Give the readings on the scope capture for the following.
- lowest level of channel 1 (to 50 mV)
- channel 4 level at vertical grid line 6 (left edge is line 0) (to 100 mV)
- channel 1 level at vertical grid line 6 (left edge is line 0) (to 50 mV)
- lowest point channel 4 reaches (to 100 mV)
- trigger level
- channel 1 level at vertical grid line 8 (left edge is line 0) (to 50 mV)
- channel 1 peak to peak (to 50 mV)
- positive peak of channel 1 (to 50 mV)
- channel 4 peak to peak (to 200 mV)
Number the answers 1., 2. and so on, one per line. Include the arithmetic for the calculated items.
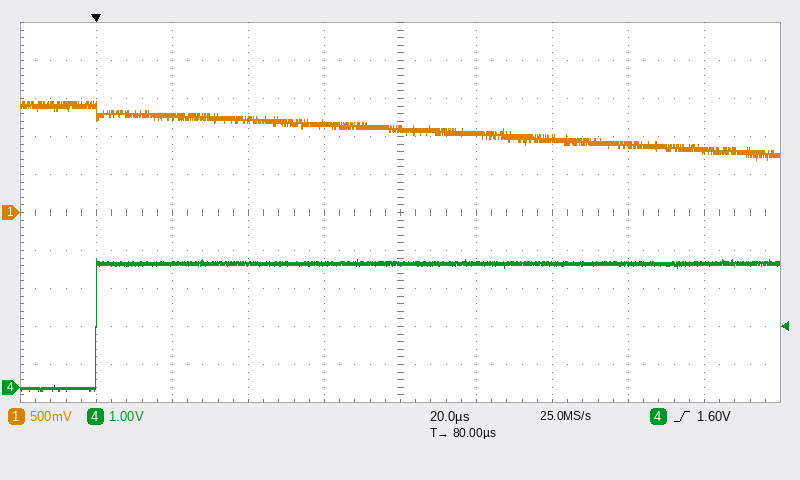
1. 700 mV
2. 3.3 V
3. 1.05 V
4. -100 mV
5. 1.60 V
6. 900 mV
7. 1.45 V − (700 mV) = 750 mV
8. 1.45 V
9. 3.4 V
